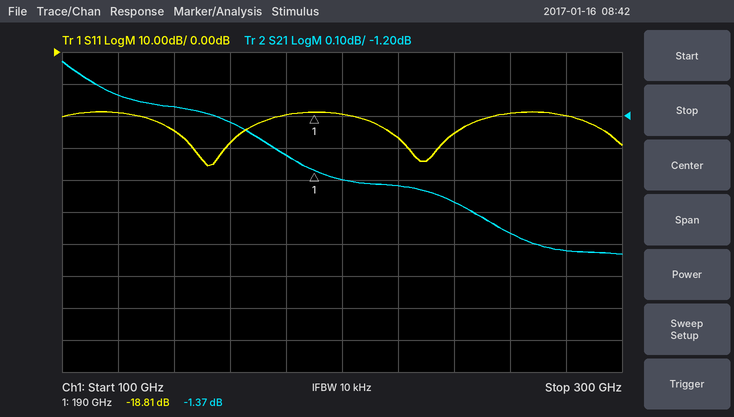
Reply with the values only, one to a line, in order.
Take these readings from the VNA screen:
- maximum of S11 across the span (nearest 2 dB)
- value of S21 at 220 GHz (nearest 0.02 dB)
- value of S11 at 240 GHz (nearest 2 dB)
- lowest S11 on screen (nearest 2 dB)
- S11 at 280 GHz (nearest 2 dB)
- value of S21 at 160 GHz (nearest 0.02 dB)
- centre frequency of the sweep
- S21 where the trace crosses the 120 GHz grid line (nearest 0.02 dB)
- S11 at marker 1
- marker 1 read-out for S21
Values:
-18 dB
-1.42 dB
-26 dB
-36 dB
-20 dB
-1.22 dB
200 GHz
-1.14 dB
-18.81 dB
-1.37 dB
